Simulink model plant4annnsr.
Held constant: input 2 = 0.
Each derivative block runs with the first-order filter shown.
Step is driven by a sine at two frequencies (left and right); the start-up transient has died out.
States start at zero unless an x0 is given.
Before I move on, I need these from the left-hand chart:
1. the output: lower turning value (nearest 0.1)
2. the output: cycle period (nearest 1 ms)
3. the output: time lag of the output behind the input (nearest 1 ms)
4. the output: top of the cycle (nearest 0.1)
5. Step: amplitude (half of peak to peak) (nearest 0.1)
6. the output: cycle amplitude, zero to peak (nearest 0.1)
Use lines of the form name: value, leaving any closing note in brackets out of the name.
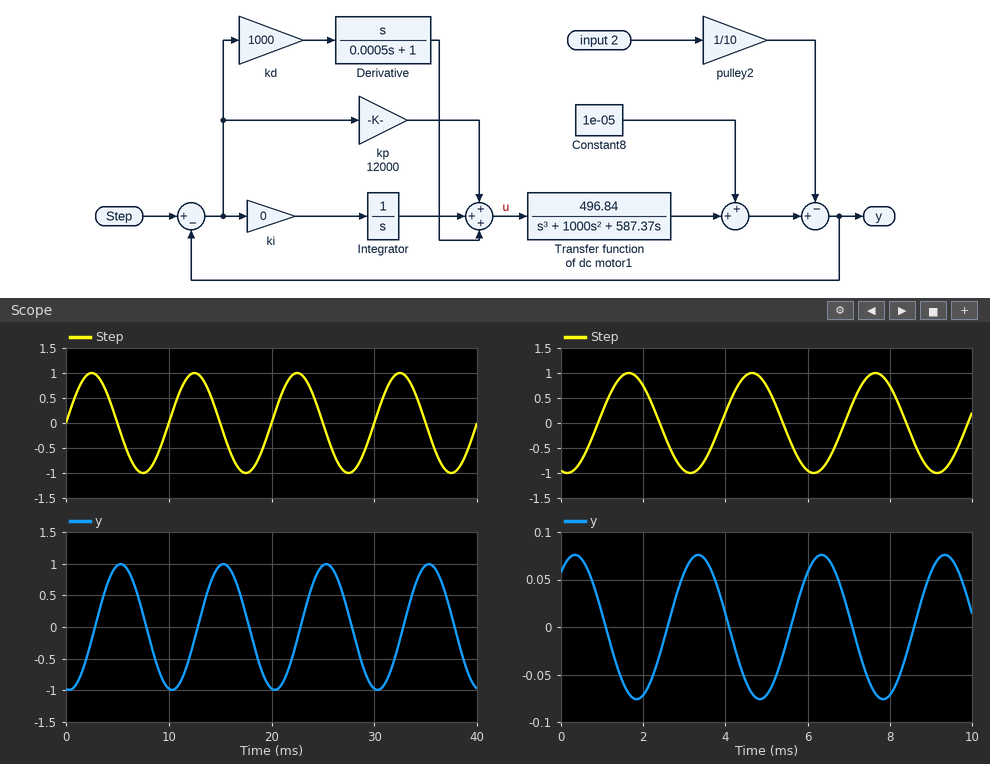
the output: lower turning value: -1.0
the output: cycle period: 10 ms
the output: time lag of the output behind the input: 3 ms
the output: top of the cycle: 1.0
Step: amplitude (half of peak to peak): 1.0
the output: cycle amplitude, zero to peak: 1.0
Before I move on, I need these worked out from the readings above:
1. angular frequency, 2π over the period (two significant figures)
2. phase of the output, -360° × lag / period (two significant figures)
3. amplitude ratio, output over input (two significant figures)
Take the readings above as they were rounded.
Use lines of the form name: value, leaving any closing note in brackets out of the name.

angular frequency, 2π over the period: 0.63 rad/ms
phase of the output, -360° × lag / period: -110°
amplitude ratio, output over input: 1.0
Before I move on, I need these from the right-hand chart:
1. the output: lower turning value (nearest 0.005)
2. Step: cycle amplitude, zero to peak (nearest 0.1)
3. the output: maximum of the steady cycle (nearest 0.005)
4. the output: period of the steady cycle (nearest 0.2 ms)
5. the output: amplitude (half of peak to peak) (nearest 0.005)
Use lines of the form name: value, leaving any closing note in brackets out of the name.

the output: lower turning value: -0.075
Step: cycle amplitude, zero to peak: 1.0
the output: maximum of the steady cycle: 0.075
the output: period of the steady cycle: 3.0 ms
the output: amplitude (half of peak to peak): 0.075
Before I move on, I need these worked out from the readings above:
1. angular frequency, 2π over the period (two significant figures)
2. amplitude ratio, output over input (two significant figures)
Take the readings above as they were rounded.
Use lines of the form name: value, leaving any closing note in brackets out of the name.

angular frequency, 2π over the period: 2.1 rad/ms
amplitude ratio, output over input: 0.075
